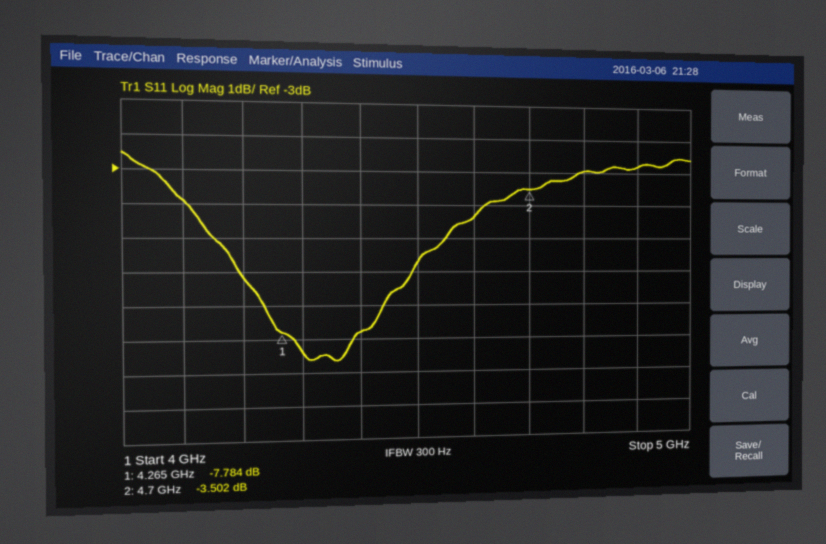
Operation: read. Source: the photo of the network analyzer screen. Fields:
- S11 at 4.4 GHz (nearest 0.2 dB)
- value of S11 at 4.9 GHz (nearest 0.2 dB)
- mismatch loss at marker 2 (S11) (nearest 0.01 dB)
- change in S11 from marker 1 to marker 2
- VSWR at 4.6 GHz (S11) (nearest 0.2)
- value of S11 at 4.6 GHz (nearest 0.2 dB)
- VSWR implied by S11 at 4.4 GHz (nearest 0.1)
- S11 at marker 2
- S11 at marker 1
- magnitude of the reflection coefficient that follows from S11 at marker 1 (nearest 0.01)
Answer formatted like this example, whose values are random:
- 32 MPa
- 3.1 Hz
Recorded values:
- -7.8 dB
- -2.8 dB
- 2.57 dB
- 4.282 dB
- 4.0
- -4.4 dB
- 2.4
- -3.502 dB
- -7.784 dB
- 0.41
